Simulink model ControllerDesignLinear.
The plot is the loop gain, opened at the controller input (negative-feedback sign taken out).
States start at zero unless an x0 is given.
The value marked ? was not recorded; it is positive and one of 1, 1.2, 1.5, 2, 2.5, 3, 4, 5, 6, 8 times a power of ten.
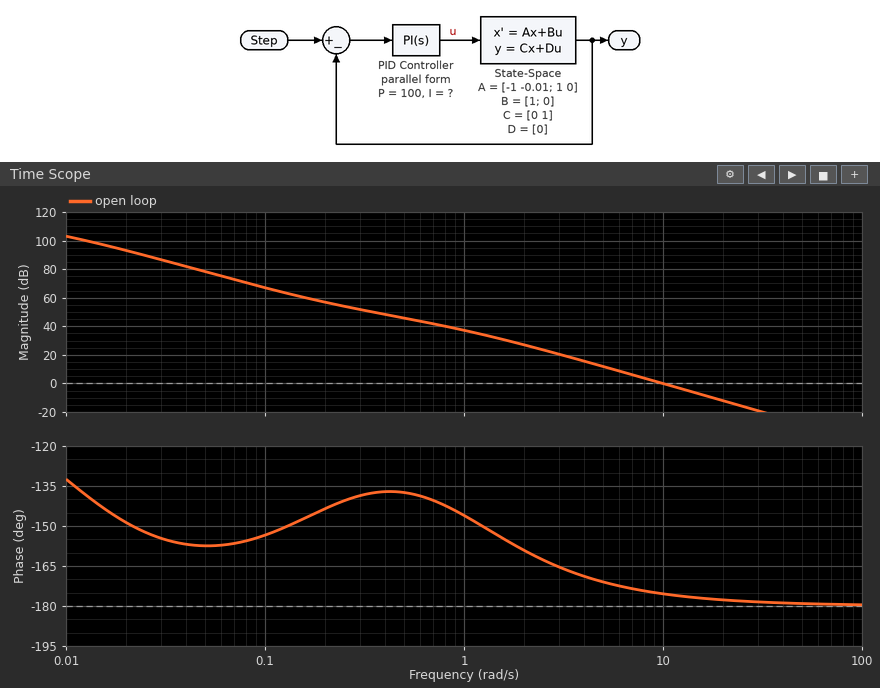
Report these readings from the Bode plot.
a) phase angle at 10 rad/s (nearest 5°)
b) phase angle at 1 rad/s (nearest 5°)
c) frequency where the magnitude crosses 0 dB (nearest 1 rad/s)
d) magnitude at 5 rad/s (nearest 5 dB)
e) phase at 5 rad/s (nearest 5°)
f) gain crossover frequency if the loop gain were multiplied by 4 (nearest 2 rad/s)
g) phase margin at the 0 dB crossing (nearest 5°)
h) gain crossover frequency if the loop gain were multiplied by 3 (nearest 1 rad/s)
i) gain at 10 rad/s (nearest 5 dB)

-175°
-145°
10 rad/s
10 dB
-170°
20 rad/s
5°
17 rad/s
0 dB
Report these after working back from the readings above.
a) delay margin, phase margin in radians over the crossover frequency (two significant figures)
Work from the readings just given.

0.0087 s
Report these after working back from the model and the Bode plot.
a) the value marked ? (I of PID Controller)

20
